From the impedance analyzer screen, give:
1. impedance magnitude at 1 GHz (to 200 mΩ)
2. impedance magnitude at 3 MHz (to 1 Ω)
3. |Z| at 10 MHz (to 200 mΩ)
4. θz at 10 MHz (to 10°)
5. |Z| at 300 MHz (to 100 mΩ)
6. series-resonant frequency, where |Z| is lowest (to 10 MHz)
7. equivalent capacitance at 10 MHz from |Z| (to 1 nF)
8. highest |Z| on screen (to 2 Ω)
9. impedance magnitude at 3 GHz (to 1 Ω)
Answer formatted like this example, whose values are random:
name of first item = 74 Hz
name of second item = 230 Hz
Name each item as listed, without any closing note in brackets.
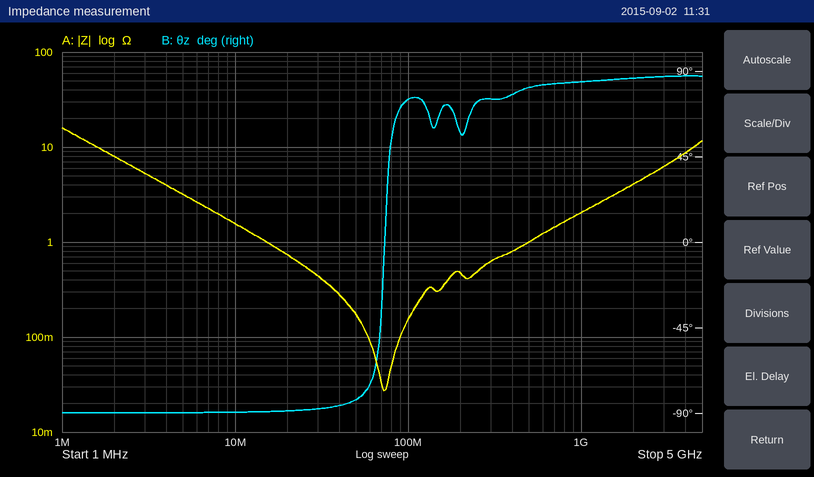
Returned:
impedance magnitude at 1 GHz = 2.0 Ω
impedance magnitude at 3 MHz = 5 Ω
|Z| at 10 MHz = 1.6 Ω
θz at 10 MHz = -90°
|Z| at 300 MHz = 600 mΩ
series-resonant frequency, where |Z| is lowest = 70 MHz
equivalent capacitance at 10 MHz from |Z| = 10 nF
highest |Z| on screen = 16 Ω
impedance magnitude at 3 GHz = 6 Ω
